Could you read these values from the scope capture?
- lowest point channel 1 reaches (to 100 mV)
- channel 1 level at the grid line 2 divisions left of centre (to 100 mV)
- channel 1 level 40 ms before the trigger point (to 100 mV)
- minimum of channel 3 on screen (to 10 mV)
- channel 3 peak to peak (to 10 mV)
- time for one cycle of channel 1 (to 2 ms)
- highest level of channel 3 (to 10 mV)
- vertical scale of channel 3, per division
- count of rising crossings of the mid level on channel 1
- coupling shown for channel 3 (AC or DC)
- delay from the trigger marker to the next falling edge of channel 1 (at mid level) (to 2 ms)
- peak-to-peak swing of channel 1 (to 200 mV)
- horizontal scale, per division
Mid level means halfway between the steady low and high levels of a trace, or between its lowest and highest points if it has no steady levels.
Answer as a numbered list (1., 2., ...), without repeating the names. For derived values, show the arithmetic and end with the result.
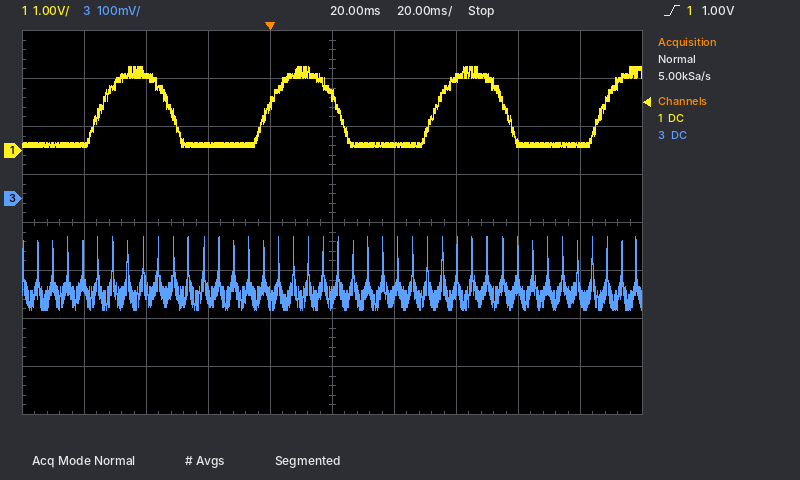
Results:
1. 100 mV
2. 100 mV
3. 1.6 V
4. -230 mV
5. -80 mV − (-230 mV) = 150 mV
6. 54 ms
7. -80 mV
8. 100 mV
9. 4
10. DC
11. 22 ms
12. 1.6 V
13. 20 ms
